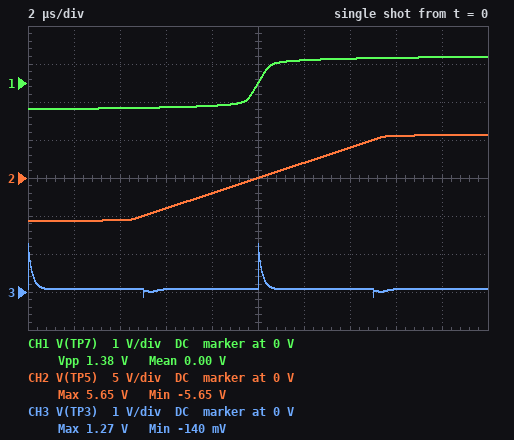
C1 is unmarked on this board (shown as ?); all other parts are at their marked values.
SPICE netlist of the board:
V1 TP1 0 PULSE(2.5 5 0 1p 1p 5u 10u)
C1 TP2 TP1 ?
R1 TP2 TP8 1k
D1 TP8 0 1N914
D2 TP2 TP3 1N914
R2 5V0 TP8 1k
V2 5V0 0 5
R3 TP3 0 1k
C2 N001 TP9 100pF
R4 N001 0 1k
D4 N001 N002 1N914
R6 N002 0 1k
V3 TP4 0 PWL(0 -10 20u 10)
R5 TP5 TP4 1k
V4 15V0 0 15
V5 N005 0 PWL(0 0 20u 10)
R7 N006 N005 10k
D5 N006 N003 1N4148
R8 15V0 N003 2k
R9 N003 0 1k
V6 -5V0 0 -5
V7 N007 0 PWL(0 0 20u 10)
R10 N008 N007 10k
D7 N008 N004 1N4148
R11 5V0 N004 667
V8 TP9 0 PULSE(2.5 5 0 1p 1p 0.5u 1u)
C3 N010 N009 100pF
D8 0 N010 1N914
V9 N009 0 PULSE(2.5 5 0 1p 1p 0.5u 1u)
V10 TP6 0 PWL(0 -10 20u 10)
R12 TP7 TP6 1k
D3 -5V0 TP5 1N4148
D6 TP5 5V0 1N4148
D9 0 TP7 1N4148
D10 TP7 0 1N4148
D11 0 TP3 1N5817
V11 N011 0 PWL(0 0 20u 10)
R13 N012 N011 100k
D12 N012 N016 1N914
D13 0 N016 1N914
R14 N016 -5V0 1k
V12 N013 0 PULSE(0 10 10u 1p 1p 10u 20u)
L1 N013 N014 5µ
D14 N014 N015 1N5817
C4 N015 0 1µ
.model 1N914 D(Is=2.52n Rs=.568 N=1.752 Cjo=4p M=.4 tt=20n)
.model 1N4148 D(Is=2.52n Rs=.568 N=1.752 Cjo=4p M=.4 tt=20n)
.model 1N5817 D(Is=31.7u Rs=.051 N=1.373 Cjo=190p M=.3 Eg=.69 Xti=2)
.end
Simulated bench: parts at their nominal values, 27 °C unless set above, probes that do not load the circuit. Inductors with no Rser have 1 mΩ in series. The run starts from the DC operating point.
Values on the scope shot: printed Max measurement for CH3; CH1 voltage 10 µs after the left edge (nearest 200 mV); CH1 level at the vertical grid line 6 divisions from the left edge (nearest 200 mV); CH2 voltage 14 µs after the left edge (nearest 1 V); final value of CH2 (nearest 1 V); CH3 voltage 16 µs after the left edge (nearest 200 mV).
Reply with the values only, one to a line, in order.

1.27 V
0 V
600 mV
4 V
6 V
0 V
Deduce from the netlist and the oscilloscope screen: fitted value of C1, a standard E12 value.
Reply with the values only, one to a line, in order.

180 pF
